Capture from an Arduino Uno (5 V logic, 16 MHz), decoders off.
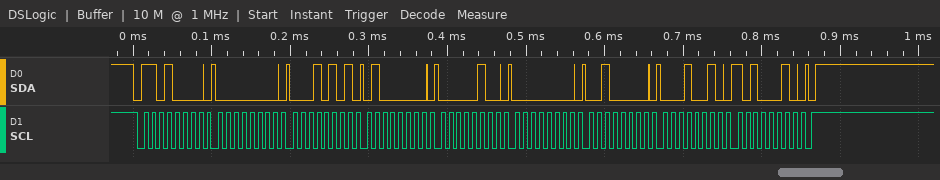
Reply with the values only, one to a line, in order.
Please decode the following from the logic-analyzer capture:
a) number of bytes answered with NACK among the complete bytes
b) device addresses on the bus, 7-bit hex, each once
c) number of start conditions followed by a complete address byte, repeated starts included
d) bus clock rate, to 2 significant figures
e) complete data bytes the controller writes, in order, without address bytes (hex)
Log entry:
0
0x68
1
100 kHz
00 15 40 04 00 20 12 A2
